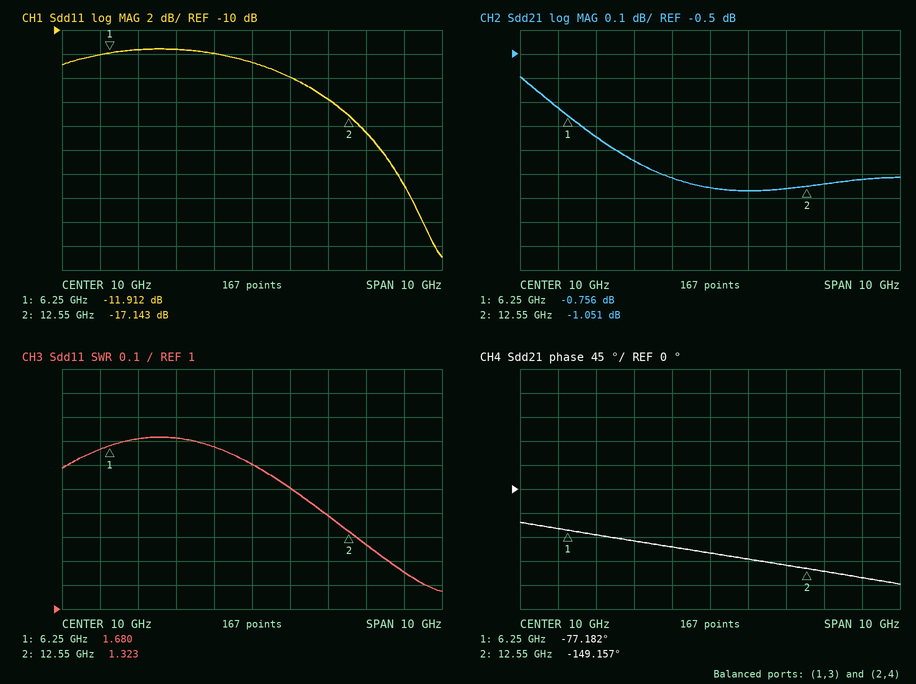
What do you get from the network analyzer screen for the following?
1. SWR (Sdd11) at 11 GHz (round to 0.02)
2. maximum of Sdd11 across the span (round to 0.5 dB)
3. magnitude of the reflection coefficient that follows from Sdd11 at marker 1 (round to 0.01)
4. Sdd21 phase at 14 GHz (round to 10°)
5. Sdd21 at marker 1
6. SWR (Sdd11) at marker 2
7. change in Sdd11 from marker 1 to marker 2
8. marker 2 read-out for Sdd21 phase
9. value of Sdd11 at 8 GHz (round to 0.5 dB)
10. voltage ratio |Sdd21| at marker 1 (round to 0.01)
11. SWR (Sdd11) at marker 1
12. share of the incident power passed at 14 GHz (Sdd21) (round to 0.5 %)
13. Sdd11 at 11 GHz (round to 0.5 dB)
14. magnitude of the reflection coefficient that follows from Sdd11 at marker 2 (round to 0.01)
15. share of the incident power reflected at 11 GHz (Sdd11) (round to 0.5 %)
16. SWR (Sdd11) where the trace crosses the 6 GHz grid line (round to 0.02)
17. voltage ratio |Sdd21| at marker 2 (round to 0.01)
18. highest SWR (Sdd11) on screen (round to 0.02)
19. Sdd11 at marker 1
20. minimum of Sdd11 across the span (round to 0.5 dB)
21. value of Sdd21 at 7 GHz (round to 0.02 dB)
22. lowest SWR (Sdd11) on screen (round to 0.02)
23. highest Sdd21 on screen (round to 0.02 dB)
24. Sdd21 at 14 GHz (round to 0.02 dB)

1.50
-11.5 dB
0.25
-170°
-0.756 dB
1.323
-5.231 dB
-149.157°
-11.5 dB
0.92
1.680
79.0 %
-14.0 dB
0.14
4.0 %
1.66
0.89
1.72
-11.912 dB
-29.0 dB
-0.84 dB
1.08
-0.60 dB
-1.02 dB
